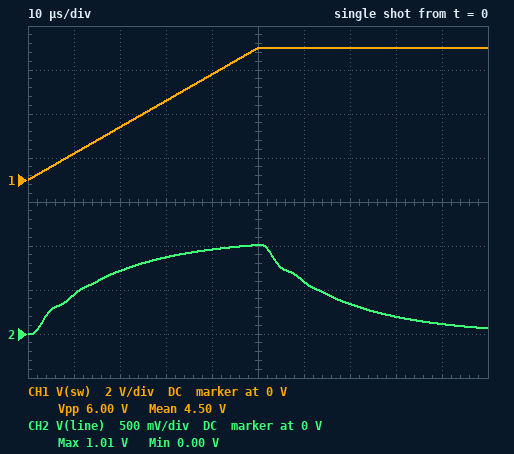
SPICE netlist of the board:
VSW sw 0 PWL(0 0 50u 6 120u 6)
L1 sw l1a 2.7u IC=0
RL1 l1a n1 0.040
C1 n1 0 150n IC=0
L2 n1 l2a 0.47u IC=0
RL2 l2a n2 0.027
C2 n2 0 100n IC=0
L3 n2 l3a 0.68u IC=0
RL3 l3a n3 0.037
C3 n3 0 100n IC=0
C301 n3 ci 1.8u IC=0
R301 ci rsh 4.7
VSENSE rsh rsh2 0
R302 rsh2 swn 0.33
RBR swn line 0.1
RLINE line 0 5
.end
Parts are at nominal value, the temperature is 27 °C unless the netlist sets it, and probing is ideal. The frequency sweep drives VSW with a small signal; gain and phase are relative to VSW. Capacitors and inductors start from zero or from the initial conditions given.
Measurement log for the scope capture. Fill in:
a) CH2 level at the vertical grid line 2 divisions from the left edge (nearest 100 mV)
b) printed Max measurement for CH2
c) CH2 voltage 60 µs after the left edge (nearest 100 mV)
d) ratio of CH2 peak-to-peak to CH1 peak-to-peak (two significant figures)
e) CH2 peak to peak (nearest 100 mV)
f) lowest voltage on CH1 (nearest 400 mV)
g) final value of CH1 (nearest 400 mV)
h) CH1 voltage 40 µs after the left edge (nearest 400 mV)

700 mV
1.01 V
600 mV
0.17
1.0 V
0 V
6.0 V
4.8 V
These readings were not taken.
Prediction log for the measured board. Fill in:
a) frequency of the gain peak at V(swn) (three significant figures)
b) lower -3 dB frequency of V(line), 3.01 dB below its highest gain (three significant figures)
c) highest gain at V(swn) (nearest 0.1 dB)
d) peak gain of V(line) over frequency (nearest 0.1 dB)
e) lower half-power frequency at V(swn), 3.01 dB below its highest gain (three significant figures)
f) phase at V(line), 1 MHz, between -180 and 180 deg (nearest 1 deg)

153 kHz
122 kHz
3.8 dB
3.6 dB
122 kHz
7 deg
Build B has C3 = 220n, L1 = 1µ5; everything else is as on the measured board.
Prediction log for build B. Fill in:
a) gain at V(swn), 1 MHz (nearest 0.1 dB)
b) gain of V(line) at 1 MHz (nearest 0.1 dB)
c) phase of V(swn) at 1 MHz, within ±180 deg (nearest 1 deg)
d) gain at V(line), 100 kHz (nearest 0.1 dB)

-29.6 dB
-29.8 dB
3 deg
-2.3 dB
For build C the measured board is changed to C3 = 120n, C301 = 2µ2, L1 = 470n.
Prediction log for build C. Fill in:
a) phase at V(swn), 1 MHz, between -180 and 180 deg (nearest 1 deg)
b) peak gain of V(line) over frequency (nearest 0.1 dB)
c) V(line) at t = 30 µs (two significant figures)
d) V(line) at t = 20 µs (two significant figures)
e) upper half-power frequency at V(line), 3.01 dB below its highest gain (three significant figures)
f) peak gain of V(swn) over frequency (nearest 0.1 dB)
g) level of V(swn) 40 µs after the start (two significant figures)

9 deg
7.0 dB
970 mV
780 mV
739 kHz
7.2 dB
1.1 V
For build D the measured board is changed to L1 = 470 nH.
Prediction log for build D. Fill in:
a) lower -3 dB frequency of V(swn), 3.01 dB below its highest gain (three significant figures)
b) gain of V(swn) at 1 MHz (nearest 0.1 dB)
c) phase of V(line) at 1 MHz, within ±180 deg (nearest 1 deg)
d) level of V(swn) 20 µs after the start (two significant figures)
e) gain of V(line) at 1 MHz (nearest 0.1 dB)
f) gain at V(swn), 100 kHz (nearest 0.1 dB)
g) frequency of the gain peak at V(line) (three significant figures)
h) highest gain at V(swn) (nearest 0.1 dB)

260 kHz
-12.2 dB
11 deg
730 mV
-12.4 dB
-4.9 dB
310 kHz
6.4 dB
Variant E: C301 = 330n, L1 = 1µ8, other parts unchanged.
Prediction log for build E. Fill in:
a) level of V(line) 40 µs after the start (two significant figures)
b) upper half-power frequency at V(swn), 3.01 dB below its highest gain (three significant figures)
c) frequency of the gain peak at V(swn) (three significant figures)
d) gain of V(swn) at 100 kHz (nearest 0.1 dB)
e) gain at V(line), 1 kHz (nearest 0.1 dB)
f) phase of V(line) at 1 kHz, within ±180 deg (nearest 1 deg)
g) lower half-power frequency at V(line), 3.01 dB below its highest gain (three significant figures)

200 mV
209 kHz
180 kHz
-3.2 dB
-39.7 dB
89 deg
148 kHz
